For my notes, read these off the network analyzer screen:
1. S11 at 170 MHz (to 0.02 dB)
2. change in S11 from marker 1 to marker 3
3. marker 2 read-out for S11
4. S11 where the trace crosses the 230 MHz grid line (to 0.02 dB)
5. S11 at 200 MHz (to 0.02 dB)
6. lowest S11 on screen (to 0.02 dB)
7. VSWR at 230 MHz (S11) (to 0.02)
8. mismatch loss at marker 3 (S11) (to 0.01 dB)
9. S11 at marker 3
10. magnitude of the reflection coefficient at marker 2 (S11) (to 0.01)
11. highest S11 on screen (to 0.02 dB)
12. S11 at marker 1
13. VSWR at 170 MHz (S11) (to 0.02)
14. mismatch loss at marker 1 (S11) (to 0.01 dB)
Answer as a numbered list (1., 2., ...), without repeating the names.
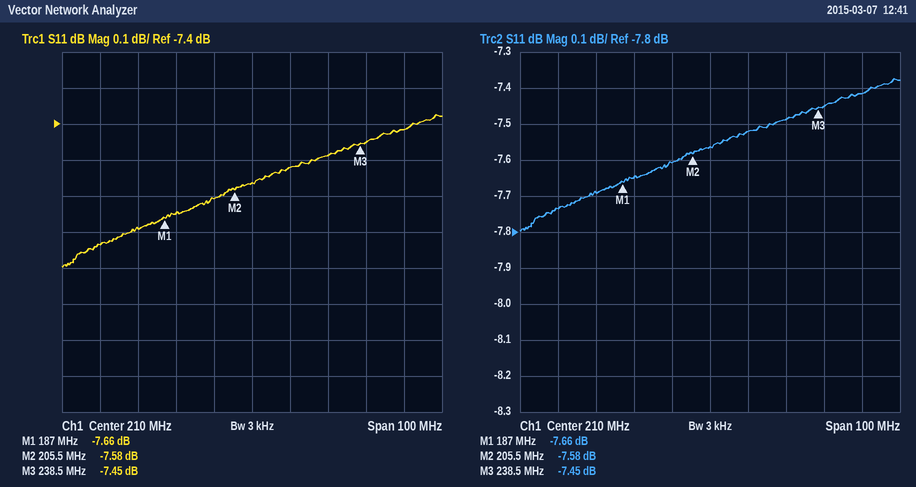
1. -7.74 dB
2. 0.21 dB
3. -7.58 dB
4. -7.48 dB
5. -7.60 dB
6. -7.80 dB
7. 2.46
8. 0.86 dB
9. -7.45 dB
10. 0.42
11. -7.38 dB
12. -7.66 dB
13. 2.40
14. 0.82 dB
